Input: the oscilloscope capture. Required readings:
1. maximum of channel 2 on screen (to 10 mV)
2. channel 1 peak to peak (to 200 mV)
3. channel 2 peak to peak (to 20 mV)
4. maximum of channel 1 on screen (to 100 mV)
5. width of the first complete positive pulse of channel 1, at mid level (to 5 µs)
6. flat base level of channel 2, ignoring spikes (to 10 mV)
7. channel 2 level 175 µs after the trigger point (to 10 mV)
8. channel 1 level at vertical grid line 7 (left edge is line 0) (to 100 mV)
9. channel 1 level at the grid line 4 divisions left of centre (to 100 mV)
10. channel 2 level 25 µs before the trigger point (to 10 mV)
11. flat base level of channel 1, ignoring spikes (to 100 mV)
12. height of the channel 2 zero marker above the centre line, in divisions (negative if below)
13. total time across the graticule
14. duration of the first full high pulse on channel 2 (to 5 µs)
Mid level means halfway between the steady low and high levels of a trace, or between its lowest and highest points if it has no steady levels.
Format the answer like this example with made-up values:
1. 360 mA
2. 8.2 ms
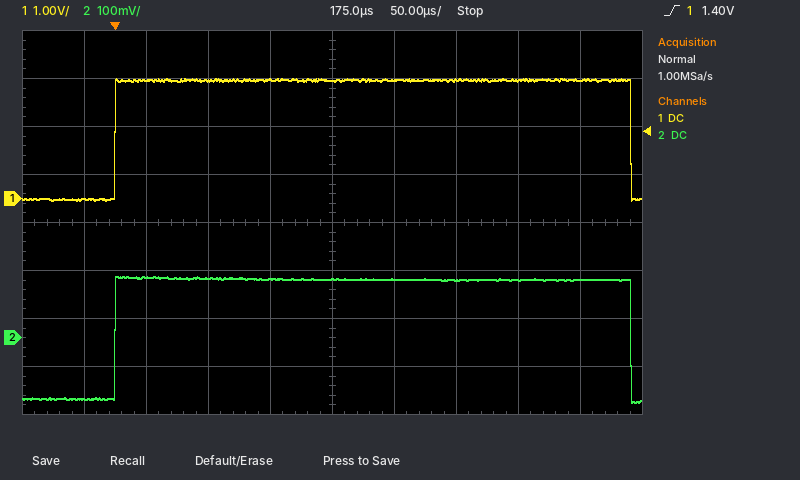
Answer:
1. 130 mV
2. 2.6 V
3. 260 mV
4. 2.5 V
5. 415 µs
6. -130 mV
7. 120 mV
8. 2.5 V
9. 0.0 V
10. -130 mV
11. 0.0 V
12. -2.4 div
13. 500 µs
14. 415 µs
